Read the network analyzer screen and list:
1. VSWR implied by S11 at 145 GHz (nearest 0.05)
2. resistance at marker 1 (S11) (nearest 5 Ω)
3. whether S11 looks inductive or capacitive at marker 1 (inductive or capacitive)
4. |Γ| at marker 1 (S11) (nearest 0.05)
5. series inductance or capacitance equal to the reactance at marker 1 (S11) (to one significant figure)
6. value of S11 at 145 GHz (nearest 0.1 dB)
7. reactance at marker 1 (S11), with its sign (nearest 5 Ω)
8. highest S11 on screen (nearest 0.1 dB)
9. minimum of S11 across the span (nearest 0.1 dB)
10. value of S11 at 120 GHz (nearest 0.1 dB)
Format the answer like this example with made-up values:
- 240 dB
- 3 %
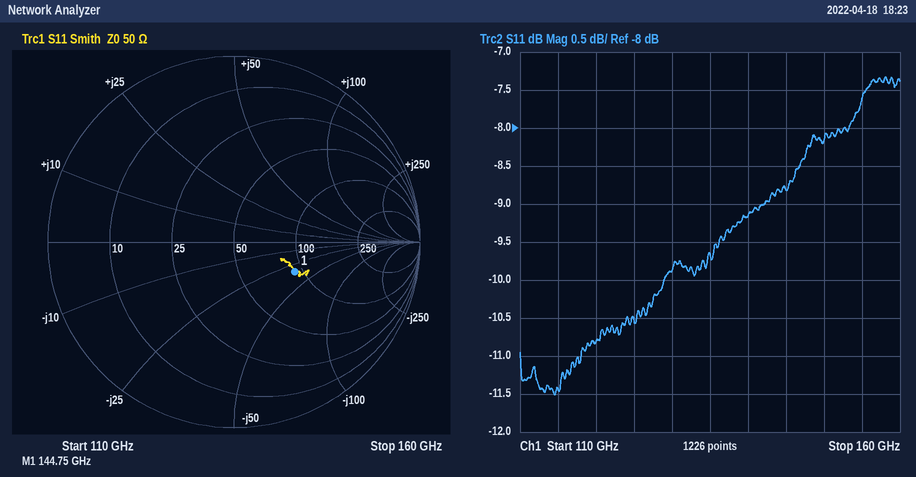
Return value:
- 2.15
- 90 Ω
- capacitive
- 0.35
- 30 fF
- -8.8 dB
- -35 Ω
- -7.3 dB
- -11.5 dB
- -10.8 dB
